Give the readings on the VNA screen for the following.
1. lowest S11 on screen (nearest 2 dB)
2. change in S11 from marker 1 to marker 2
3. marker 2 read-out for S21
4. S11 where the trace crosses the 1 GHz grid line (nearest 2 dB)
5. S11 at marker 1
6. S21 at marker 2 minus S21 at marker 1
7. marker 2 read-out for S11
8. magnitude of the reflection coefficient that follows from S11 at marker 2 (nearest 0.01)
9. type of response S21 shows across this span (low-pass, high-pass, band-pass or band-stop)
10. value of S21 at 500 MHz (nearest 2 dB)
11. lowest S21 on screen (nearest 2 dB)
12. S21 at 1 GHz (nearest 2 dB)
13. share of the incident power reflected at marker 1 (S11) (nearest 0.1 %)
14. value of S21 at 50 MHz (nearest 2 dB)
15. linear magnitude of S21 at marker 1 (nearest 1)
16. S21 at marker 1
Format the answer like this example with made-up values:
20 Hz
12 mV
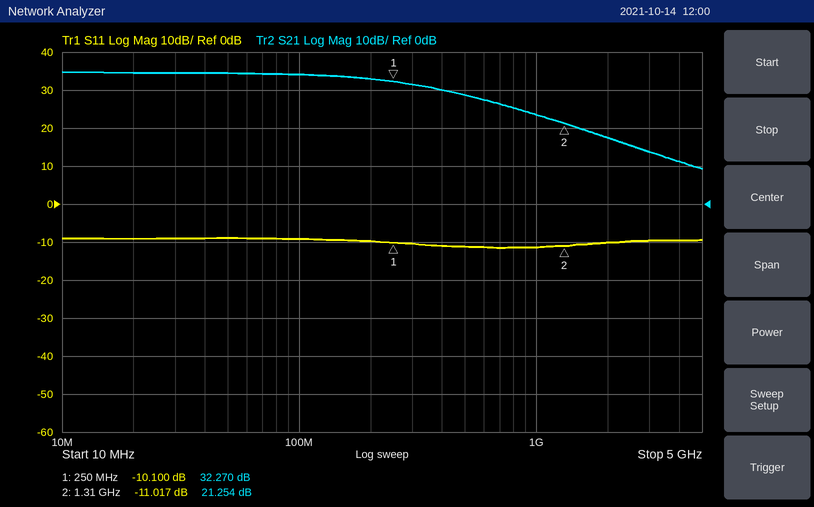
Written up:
-12 dB
-0.917 dB
21.254 dB
-12 dB
-10.100 dB
-11.016 dB
-11.017 dB
0.28
low-pass
28 dB
10 dB
24 dB
9.8 %
34 dB
41
32.270 dB
